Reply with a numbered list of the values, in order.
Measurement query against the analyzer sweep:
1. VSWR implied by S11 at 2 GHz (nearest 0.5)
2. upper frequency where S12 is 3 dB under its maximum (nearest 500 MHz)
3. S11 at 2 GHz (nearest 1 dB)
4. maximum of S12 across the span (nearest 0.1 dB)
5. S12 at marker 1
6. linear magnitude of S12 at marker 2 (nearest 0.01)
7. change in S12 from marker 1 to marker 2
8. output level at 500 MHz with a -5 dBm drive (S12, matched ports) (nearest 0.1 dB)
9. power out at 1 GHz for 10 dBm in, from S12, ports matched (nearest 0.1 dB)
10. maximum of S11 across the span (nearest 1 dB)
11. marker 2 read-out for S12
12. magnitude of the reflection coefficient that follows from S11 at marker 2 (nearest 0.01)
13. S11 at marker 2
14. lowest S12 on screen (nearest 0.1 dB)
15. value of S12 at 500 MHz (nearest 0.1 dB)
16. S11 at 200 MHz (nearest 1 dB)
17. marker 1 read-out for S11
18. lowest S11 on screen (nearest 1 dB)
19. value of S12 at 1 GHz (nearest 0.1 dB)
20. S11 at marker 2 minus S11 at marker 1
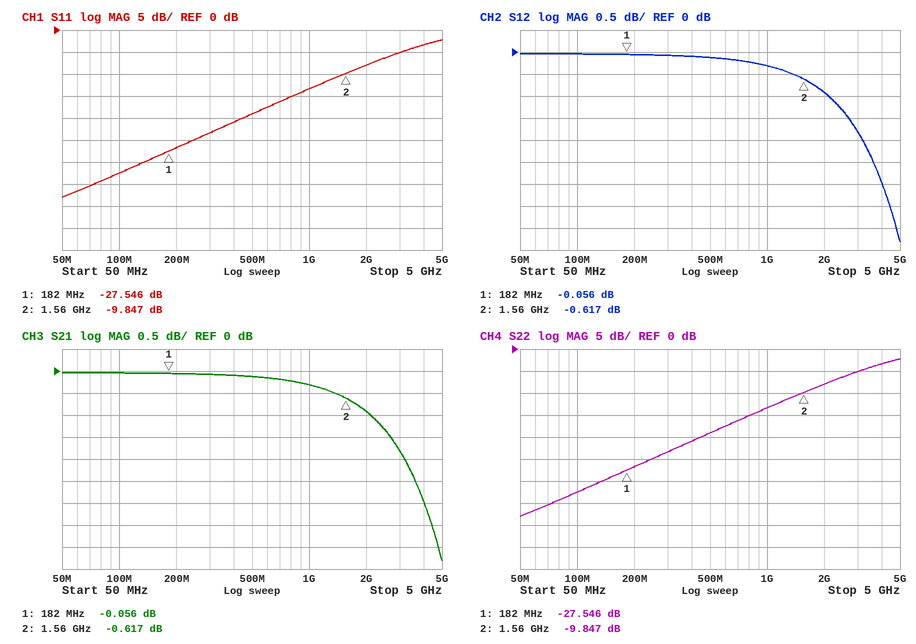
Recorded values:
1. 2.5
2. 4.0 GHz
3. -8 dB
4. 0.0 dB
5. -0.056 dB
6. 0.93
7. -0.561 dB
8. -5.1 dBm
9. 9.7 dBm
10. -2 dB
11. -0.617 dB
12. 0.32
13. -9.847 dB
14. -4.3 dB
15. -0.1 dB
16. -27 dB
17. -27.546 dB
18. -38 dB
19. -0.3 dB
20. 17.699 dB
